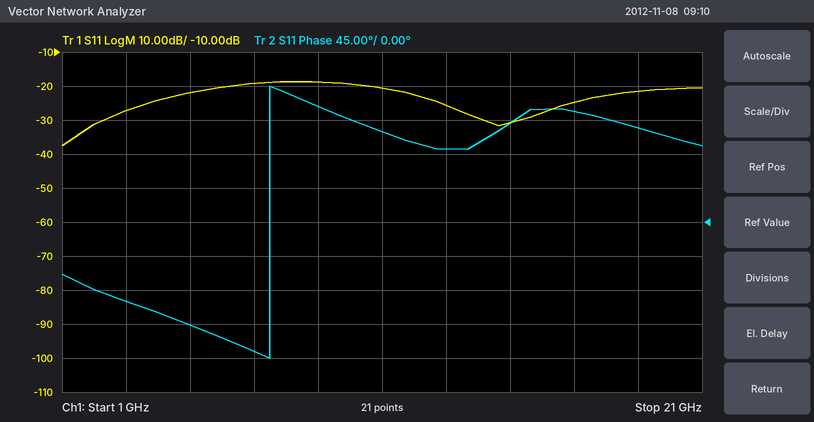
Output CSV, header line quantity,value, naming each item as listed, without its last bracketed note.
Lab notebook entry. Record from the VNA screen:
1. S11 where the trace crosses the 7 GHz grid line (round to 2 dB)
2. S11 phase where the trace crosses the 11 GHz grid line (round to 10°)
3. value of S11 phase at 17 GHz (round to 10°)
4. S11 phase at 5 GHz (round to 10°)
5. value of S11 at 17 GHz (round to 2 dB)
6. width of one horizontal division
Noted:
quantity,value
S11 where the trace crosses the 7 GHz grid line,-20 dB
S11 phase where the trace crosses the 11 GHz grid line,120°
value of S11 phase at 17 GHz,150°
S11 phase at 5 GHz,-140°
value of S11 at 17 GHz,-24 dB
width of one horizontal division,2 GHz
